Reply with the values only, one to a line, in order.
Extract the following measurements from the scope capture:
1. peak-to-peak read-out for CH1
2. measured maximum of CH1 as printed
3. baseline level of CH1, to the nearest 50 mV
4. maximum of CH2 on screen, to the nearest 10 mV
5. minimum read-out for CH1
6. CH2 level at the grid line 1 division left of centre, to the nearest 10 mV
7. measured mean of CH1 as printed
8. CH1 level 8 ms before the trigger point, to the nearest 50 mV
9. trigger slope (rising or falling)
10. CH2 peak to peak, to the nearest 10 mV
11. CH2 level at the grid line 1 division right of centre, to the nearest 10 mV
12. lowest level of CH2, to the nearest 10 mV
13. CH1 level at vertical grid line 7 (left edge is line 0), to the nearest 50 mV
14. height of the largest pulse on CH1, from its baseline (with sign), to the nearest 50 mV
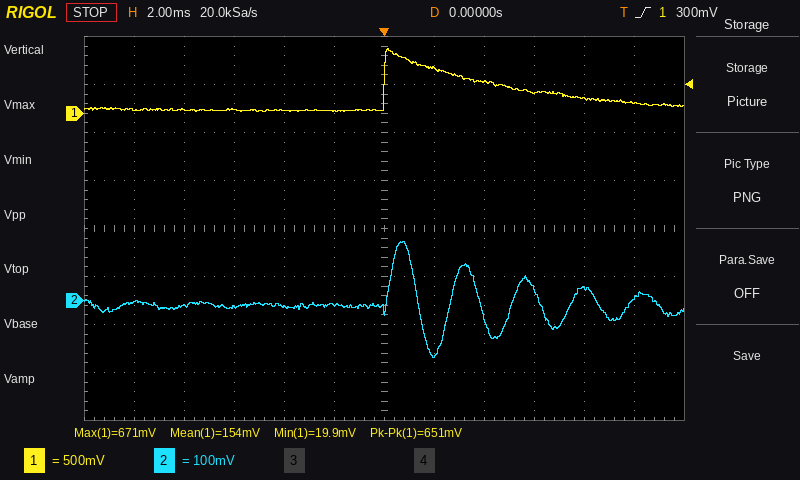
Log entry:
651 mV
671 mV
50 mV
120 mV
19.9 mV
-10 mV
154 mV
50 mV
rising
240 mV
-110 mV
-120 mV
450 mV
+650 mV
